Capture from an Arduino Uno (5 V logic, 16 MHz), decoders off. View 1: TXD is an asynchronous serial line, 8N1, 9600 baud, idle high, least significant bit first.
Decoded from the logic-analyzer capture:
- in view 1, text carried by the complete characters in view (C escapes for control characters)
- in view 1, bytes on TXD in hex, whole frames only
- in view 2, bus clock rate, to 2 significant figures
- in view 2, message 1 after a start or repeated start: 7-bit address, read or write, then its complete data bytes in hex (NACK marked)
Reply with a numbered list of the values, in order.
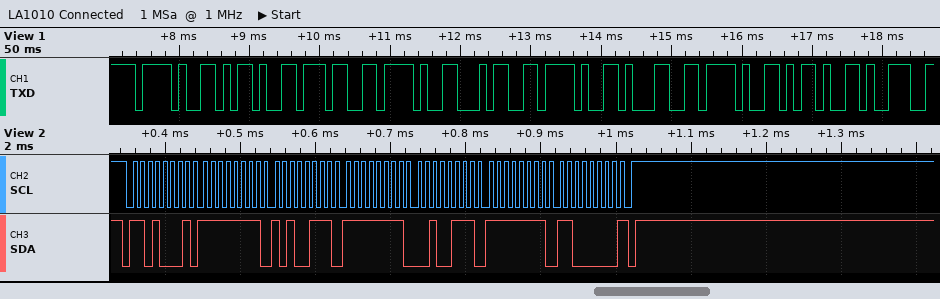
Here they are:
1. "/-7/4/1/-9"
2. 2F 2D 37 2F 34 2F 31 2F 2D 39
3. 100 kHz
4. 0x68 read: FF A7 FF 27 FF C0 NACK
